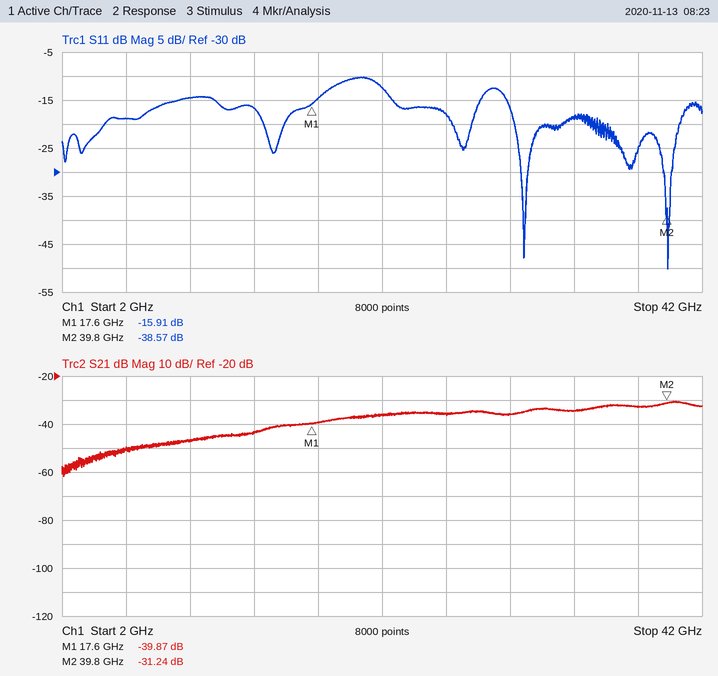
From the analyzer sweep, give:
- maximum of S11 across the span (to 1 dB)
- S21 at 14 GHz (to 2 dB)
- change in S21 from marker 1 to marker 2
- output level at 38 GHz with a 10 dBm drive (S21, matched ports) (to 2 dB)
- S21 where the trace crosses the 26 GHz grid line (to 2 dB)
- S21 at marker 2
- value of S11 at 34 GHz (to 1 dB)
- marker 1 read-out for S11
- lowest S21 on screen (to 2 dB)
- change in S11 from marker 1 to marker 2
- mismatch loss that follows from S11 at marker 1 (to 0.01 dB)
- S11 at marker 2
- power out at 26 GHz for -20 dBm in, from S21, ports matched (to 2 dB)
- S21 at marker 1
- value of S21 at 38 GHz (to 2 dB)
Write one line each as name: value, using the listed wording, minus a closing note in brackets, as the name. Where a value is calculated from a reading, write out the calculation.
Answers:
maximum of S11 across the span: -10 dB
S21 at 14 GHz: -44 dB
change in S21 from marker 1 to marker 2: -31.24 − (-39.87) = 8.63 dB
output level at 38 GHz with a 10 dBm drive (S21, matched ports): 10 dBm + (-32 dB) = -22 dBm
S21 where the trace crosses the 26 GHz grid line: -36 dB
S21 at marker 2: -31.24 dB
value of S11 at 34 GHz: -19 dB
marker 1 read-out for S11: -15.91 dB
lowest S21 on screen: -62 dB
change in S11 from marker 1 to marker 2: -38.57 − (-15.91) = -22.66 dB
mismatch loss that follows from S11 at marker 1: −10 log10(1 − 10^(-15.91/10)) ≈ 0.11 dB
S11 at marker 2: -38.57 dB
power out at 26 GHz for -20 dBm in, from S21, ports matched: -20 dBm + (-36 dB) = -56 dBm
S21 at marker 1: -39.87 dB
value of S21 at 38 GHz: -32 dB
